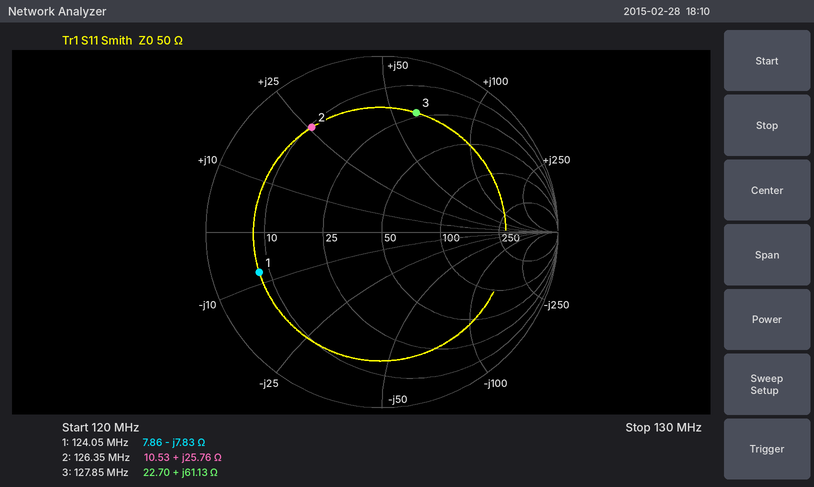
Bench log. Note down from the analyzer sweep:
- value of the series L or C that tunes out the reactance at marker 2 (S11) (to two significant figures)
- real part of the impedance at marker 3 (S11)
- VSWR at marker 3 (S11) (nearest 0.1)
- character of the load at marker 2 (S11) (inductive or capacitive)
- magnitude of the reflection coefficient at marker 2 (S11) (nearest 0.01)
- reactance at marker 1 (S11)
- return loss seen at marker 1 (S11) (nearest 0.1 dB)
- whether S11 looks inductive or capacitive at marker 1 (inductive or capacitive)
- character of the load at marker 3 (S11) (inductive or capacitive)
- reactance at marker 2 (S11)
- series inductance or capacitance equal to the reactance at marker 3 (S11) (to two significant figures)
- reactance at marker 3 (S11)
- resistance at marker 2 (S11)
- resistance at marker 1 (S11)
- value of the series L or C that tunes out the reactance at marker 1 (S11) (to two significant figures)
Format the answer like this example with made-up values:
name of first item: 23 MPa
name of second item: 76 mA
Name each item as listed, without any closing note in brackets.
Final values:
value of the series L or C that tunes out the reactance at marker 2 (S11): 49 pF
real part of the impedance at marker 3: 22.70 Ω
VSWR at marker 3 (S11): 5.8
character of the load at marker 2 (S11): inductive
magnitude of the reflection coefficient at marker 2 (S11): 0.72
reactance at marker 1: -7.83 Ω
return loss seen at marker 1 (S11): 2.7 dB
whether S11 looks inductive or capacitive at marker 1: capacitive
character of the load at marker 3 (S11): inductive
reactance at marker 2: +25.76 Ω
series inductance or capacitance equal to the reactance at marker 3 (S11): 76 nH
reactance at marker 3: +61.13 Ω
resistance at marker 2: 10.53 Ω
resistance at marker 1: 7.86 Ω
value of the series L or C that tunes out the reactance at marker 1 (S11): 10 nH
